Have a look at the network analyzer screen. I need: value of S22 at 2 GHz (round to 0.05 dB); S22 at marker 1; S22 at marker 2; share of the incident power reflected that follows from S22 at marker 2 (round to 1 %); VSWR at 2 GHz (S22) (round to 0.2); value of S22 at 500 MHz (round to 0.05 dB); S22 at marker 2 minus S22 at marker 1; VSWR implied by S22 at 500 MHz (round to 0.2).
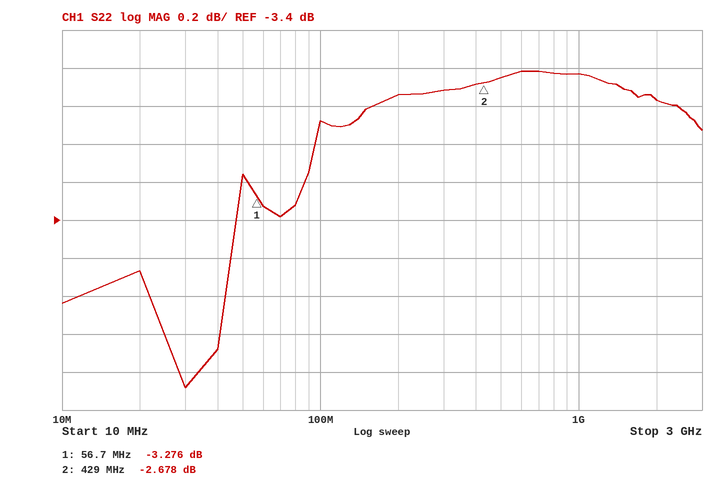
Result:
-2.75 dB
-3.276 dB
-2.678 dB
54 %
6.4
-2.65 dB
0.598 dB
6.6
